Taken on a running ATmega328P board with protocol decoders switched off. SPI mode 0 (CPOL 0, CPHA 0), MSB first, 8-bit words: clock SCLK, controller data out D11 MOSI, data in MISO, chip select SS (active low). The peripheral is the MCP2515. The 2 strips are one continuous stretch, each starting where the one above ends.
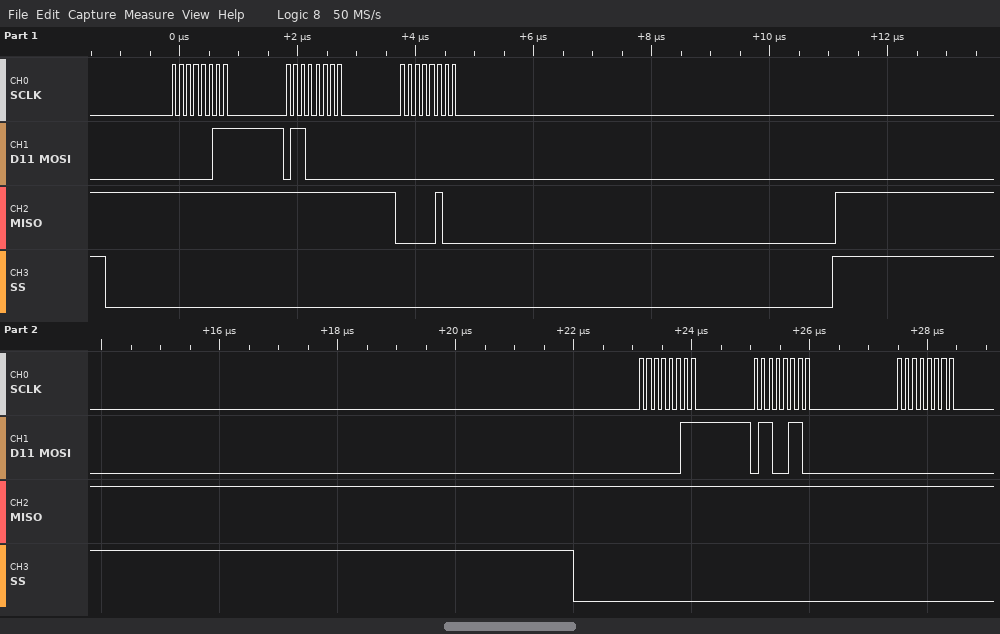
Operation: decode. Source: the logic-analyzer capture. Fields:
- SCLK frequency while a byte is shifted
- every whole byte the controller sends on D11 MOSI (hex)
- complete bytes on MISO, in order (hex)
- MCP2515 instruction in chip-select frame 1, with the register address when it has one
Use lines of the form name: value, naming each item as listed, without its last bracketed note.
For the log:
SCLK frequency while a byte is shifted: 8 MHz
every whole byte the controller sends on D11 MOSI: 0x03 0x60 0x00 0x03 0x66 0x00
complete bytes on MISO, in order: 0xFF 0xFF 0x04 0xFF 0xFF 0xFF
MCP2515 instruction in chip-select frame 1, with the register address when it has one: READ 0x60
